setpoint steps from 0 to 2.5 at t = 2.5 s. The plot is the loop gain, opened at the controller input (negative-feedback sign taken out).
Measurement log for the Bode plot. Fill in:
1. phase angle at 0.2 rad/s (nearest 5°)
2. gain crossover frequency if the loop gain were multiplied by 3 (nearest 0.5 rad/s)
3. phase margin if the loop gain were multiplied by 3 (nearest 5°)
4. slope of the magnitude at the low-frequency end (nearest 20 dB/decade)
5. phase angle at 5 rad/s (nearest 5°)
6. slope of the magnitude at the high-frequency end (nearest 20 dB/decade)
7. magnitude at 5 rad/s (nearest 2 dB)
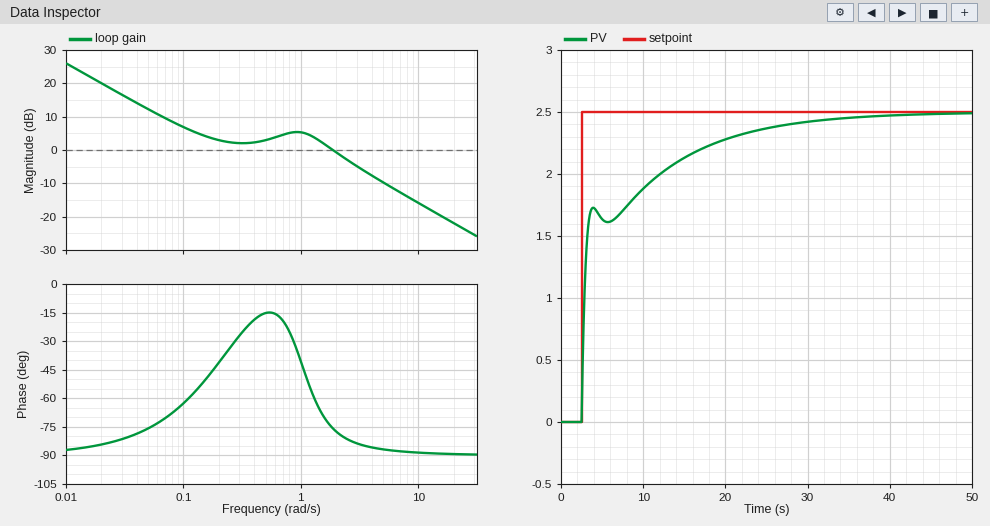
-40°
5.0 rad/s
95°
-20 dB/decade
-85°
-20 dB/decade
-10 dB
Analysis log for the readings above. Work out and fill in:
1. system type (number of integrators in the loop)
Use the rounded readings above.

1
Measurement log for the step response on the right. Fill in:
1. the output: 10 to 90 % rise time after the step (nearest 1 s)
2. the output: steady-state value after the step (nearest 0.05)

16 s
2.50
